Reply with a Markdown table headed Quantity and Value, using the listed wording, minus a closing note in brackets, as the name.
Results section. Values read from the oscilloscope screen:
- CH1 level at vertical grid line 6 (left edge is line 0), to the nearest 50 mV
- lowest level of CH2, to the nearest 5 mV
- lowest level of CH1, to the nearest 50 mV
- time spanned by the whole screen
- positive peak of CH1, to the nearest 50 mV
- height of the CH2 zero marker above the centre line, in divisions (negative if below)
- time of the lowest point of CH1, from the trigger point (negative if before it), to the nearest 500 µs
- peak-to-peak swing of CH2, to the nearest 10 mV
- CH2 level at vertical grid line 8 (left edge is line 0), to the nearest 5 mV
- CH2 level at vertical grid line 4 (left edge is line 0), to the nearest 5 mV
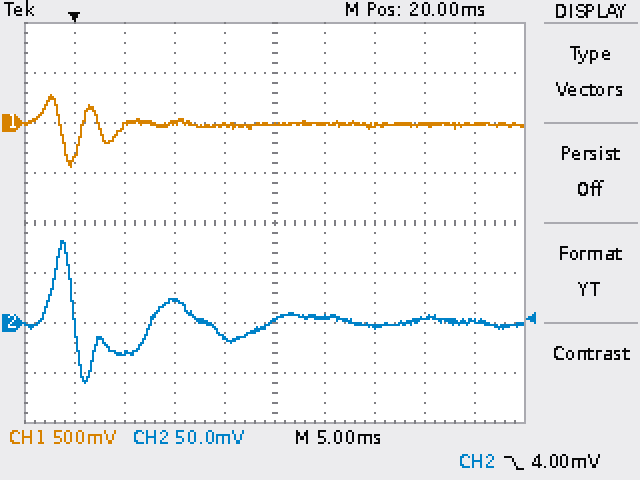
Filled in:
| Quantity | Value |
|---|---|
| CH1 level at vertical grid line 6 (left edge is line 0), to the nearest 50 mV | 0 mV |
| lowest level of CH2, to the nearest 5 mV | -60 mV |
| lowest level of CH1, to the nearest 50 mV | -450 mV |
| time spanned by the whole screen | 50 ms |
| positive peak of CH1, to the nearest 50 mV | 300 mV |
| height of the CH2 zero marker above the centre line, in divisions | -2.0 div |
| time of the lowest point of CH1, from the trigger point (negative if before it), to the nearest 500 µs | -500 µs |
| peak-to-peak swing of CH2, to the nearest 10 mV | 140 mV |
| CH2 level at vertical grid line 8 (left edge is line 0), to the nearest 5 mV | 5 mV |
| CH2 level at vertical grid line 4 (left edge is line 0), to the nearest 5 mV | -15 mV |
